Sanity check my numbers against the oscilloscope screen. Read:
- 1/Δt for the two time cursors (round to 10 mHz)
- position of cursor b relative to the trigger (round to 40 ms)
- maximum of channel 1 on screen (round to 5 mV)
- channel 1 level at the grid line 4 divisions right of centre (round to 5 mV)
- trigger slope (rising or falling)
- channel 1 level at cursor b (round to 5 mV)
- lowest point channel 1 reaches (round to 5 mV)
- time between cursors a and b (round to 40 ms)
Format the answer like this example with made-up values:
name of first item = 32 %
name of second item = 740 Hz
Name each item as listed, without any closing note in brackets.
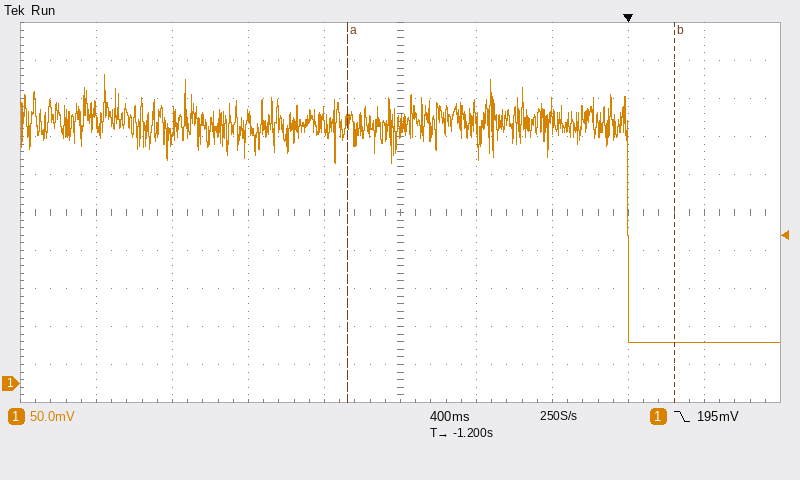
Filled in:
1/Δt for the two time cursors = 580 mHz
position of cursor b relative to the trigger = +240 ms
maximum of channel 1 on screen = 405 mV
channel 1 level at the grid line 4 divisions right of centre = 55 mV
trigger slope = falling
channel 1 level at cursor b = 55 mV
lowest point channel 1 reaches = 55 mV
time between cursors a and b = 1.72 s
